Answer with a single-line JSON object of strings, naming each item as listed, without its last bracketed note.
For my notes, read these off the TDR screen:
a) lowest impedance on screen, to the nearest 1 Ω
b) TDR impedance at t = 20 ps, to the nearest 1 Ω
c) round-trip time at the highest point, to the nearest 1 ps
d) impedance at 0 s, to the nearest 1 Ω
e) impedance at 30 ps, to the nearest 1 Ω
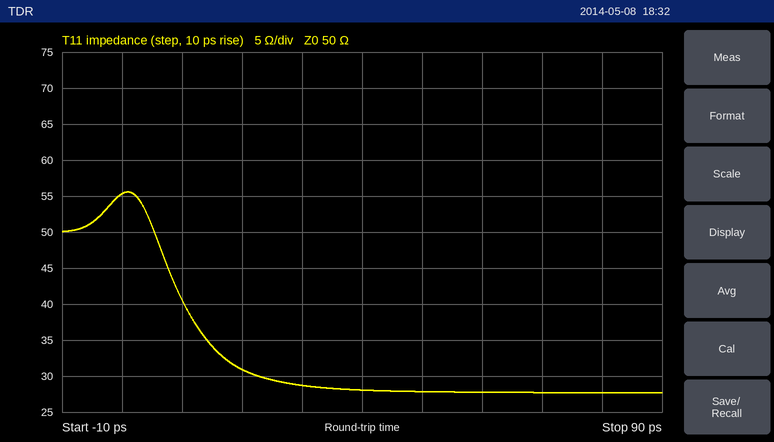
{"lowest impedance on screen, to the nearest 1 Ω": "28 Ω", "TDR impedance at t = 20 ps, to the nearest 1 Ω": "31 Ω", "round-trip time at the highest point, to the nearest 1 ps": "1 ps", "impedance at 0 s, to the nearest 1 Ω": "55 Ω", "impedance at 30 ps, to the nearest 1 Ω": "29 Ω"}
